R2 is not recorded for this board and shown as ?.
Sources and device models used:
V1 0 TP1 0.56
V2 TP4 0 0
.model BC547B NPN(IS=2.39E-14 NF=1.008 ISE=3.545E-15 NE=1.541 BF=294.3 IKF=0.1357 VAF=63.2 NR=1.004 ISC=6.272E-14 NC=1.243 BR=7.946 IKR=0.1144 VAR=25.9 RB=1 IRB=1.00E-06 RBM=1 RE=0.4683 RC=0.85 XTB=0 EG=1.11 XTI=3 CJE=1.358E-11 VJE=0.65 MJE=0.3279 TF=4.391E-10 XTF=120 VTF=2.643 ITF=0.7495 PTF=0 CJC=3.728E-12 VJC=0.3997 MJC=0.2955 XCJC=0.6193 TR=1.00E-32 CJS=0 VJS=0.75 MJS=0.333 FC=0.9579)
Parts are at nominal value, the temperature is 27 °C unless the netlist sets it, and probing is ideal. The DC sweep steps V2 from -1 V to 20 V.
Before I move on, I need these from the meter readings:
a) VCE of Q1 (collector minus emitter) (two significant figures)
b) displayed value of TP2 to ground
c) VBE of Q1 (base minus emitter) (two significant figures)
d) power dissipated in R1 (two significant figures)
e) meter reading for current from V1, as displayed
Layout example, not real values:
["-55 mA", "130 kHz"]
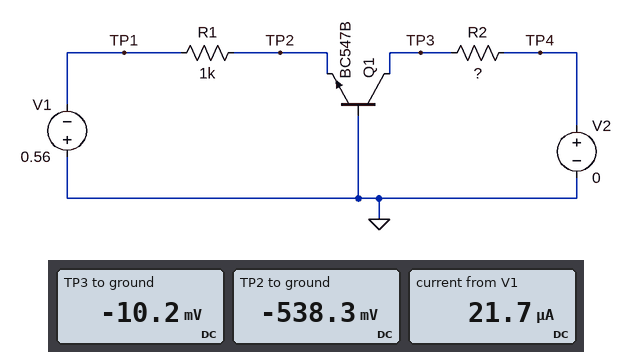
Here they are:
["530 mV", "-538.3 mV", "540 mV", "470 nW", "21.7 µA"]
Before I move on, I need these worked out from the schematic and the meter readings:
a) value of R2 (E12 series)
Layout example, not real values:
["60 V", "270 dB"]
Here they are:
["470 Ω"]
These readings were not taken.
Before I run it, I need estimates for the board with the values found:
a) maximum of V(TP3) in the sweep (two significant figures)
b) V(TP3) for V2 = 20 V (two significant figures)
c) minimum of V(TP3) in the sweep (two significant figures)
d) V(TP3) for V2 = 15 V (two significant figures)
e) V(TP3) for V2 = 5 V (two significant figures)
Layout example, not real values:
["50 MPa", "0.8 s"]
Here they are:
["20 V", "20 V", "-670 mV", "15 V", "5.0 V"]
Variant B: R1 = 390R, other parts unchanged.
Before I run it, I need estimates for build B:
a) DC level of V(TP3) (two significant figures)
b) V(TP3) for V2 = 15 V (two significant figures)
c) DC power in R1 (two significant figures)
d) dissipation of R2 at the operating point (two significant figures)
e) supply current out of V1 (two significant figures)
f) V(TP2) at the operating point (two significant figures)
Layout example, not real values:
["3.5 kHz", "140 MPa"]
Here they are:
["-15 mV", "15 V", "380 nW", "460 nW", "31 µA", "-550 mV"]
